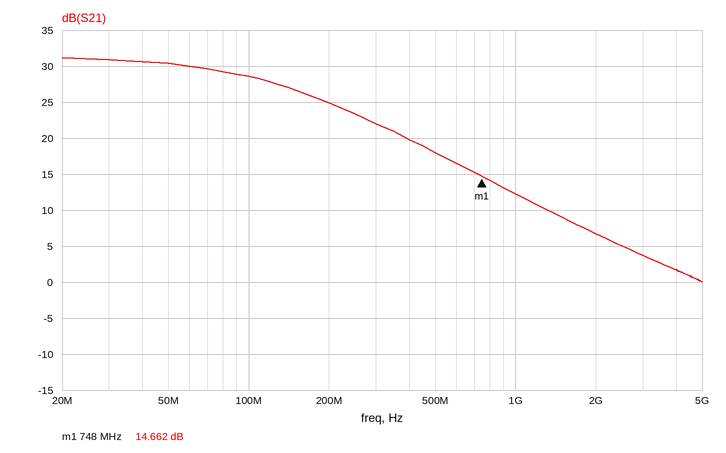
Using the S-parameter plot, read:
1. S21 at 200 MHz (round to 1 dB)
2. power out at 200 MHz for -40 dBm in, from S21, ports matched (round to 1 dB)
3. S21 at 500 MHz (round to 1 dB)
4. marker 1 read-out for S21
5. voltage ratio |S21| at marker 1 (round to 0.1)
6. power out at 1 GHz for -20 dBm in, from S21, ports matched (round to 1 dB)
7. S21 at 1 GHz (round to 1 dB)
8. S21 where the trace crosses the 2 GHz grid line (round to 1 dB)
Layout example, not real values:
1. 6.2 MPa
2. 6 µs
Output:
1. 25 dB
2. -15 dBm
3. 18 dB
4. 14.662 dB
5. 5.4
6. -8 dBm
7. 12 dB
8. 7 dB
